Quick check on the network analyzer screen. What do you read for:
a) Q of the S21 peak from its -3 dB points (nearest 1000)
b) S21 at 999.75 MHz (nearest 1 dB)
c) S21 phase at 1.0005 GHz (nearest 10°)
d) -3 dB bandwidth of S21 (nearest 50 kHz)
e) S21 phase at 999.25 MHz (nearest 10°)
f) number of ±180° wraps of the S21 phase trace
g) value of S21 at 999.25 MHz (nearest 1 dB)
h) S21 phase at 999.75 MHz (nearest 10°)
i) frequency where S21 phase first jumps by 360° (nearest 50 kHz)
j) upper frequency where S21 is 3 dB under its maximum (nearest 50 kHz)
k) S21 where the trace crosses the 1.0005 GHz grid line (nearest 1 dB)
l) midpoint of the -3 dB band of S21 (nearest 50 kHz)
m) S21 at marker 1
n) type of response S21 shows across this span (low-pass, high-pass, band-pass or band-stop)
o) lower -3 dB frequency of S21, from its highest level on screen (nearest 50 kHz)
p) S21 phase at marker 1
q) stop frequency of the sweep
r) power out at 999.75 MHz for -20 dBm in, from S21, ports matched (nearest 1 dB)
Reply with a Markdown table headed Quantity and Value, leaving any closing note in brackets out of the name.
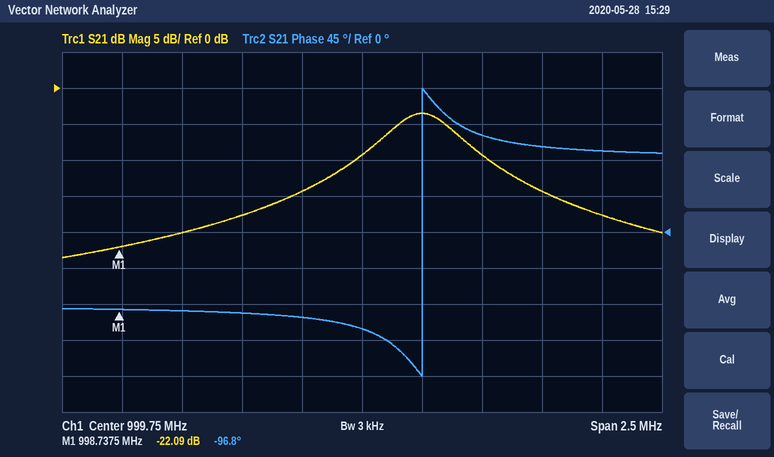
| Quantity | Value |
|---|---|
| Q of the S21 peak from its -3 dB points | 3000 |
| S21 at 999.75 MHz | -9 dB |
| S21 phase at 1.0005 GHz | 110° |
| -3 dB bandwidth of S21 | 300 kHz |
| S21 phase at 999.25 MHz | -100° |
| number of ±180° wraps of the S21 phase trace | 1 |
| value of S21 at 999.25 MHz | -18 dB |
| S21 phase at 999.75 MHz | -120° |
| frequency where S21 phase first jumps by 360° | 1.00000 GHz |
| upper frequency where S21 is 3 dB under its maximum | 1.00015 GHz |
| S21 where the trace crosses the 1.0005 GHz grid line | -14 dB |
| midpoint of the -3 dB band of S21 | 1.00000 GHz |
| S21 at marker 1 | -22.09 dB |
| type of response S21 shows across this span | band-pass |
| lower -3 dB frequency of S21, from its highest level on screen | 999.85 MHz |
| S21 phase at marker 1 | -96.8° |
| stop frequency of the sweep | 1.001 GHz |
| power out at 999.75 MHz for -20 dBm in, from S21, ports matched | -29 dBm |
